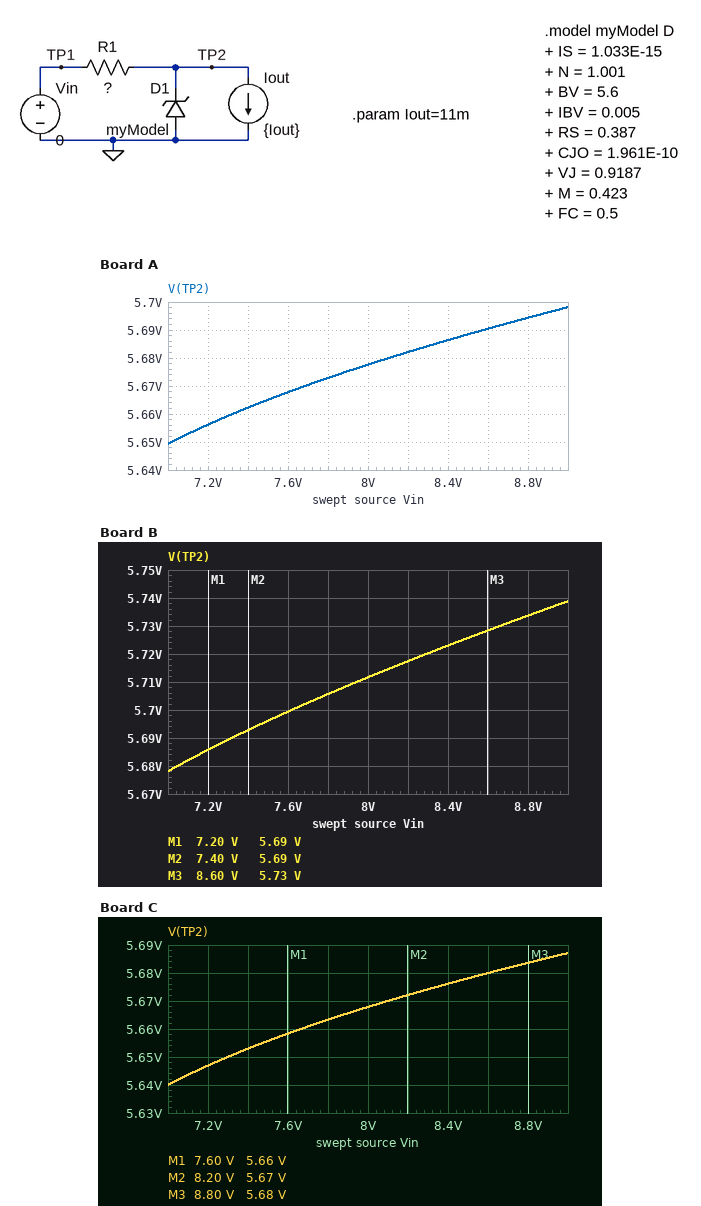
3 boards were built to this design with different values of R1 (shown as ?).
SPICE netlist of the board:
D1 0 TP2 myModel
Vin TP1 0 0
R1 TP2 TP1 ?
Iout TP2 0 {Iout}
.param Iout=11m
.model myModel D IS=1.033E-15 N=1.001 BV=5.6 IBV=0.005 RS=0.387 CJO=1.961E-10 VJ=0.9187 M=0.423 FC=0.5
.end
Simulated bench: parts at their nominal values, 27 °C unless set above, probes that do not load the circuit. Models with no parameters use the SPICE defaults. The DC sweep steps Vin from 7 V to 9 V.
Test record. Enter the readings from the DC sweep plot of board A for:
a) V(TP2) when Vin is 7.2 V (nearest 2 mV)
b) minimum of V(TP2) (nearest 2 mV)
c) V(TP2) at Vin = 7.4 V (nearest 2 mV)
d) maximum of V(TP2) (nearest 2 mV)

5.656 V
5.650 V
5.662 V
5.698 V
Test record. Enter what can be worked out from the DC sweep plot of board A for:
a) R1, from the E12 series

39 Ω
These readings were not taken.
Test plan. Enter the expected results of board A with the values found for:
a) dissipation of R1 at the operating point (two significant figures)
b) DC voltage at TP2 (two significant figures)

4.7 mW
-430 mV
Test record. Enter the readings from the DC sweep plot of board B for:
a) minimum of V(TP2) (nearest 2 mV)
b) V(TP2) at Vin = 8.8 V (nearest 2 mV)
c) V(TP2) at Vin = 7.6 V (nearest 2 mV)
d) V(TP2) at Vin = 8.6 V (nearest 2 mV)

5.678 V
5.734 V
5.700 V
5.728 V
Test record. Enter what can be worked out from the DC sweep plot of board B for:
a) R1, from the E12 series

22 Ω
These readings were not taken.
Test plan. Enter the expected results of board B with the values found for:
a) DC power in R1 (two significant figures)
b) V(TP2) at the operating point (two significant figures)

2.7 mW
-240 mV
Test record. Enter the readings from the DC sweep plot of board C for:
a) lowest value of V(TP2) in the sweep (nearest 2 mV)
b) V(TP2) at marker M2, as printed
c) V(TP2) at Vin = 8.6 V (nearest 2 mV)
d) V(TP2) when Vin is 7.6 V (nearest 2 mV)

5.640 V
5.67 V
5.680 V
5.658 V
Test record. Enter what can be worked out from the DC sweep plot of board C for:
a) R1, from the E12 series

47 Ω
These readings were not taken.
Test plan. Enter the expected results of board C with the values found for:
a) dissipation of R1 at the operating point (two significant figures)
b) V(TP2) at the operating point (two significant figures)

5.7 mW
-520 mV
